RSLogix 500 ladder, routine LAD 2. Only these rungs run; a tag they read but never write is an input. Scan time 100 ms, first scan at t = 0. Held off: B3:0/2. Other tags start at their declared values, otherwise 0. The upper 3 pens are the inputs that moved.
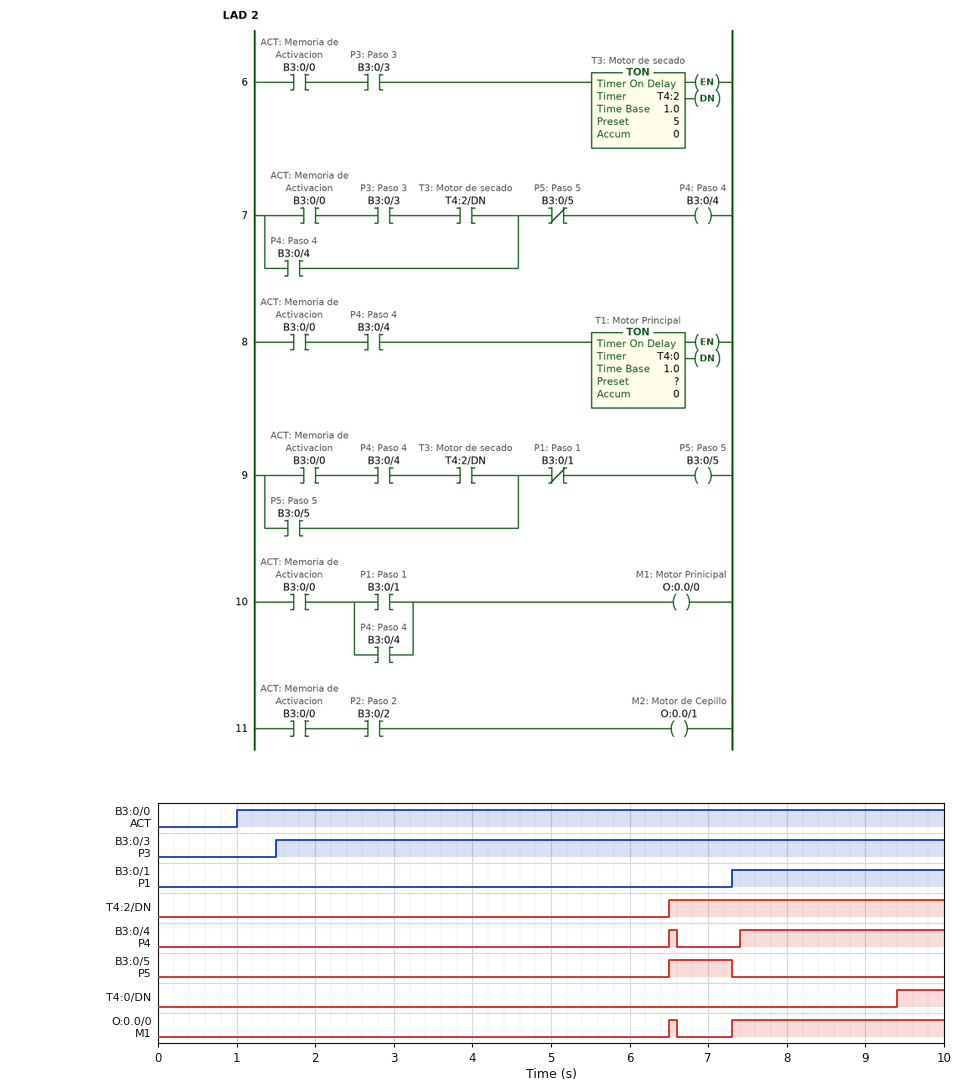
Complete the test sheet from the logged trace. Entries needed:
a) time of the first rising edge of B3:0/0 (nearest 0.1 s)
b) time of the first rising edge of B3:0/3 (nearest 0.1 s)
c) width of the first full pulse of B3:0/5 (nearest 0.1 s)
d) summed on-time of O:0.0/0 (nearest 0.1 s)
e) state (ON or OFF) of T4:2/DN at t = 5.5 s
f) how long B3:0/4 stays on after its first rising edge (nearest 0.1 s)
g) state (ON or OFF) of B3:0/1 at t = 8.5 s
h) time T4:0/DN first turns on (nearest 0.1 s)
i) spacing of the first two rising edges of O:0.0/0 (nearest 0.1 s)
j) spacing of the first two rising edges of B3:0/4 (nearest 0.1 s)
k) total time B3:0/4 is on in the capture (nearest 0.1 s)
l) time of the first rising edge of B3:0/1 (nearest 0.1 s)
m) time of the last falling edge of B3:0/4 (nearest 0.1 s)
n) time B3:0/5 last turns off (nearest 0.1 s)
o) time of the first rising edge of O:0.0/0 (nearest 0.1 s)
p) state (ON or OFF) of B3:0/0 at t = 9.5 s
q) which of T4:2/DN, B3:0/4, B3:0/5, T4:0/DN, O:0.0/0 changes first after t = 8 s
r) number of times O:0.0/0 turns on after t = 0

1.0 s
1.5 s
0.8 s
2.8 s
OFF
0.1 s
ON
9.4 s
0.8 s
0.9 s
2.7 s
7.3 s
6.6 s
7.3 s
6.5 s
ON
T4:0/DN
2
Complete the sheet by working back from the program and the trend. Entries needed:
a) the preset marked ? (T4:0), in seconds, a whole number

2 s
